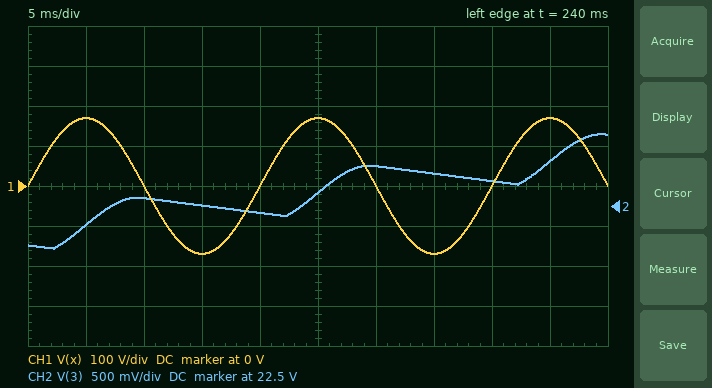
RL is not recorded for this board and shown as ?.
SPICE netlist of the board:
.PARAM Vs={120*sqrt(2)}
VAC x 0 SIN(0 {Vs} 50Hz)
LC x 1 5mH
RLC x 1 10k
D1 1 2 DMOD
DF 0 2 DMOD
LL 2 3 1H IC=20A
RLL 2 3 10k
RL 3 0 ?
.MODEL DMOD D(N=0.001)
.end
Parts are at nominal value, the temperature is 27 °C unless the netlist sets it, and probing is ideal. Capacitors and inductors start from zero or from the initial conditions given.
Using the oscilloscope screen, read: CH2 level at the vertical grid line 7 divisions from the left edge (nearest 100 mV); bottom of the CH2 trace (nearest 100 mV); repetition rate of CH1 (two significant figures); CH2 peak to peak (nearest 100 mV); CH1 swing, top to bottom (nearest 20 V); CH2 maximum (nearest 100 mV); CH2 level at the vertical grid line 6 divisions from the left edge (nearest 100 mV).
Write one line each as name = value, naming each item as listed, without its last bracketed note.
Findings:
CH2 level at the vertical grid line 7 divisions from the left edge = 22.9 V
bottom of the CH2 trace = 22.0 V
repetition rate of CH1 = 50 Hz
CH2 peak to peak = 1.4 V
CH1 swing, top to bottom = 340 V
CH2 maximum = 23.4 V
CH2 level at the vertical grid line 6 divisions from the left edge = 23.0 V
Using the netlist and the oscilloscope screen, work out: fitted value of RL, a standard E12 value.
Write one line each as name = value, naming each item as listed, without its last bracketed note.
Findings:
fitted value of RL, a standard E12 value = 0.82 Ω
